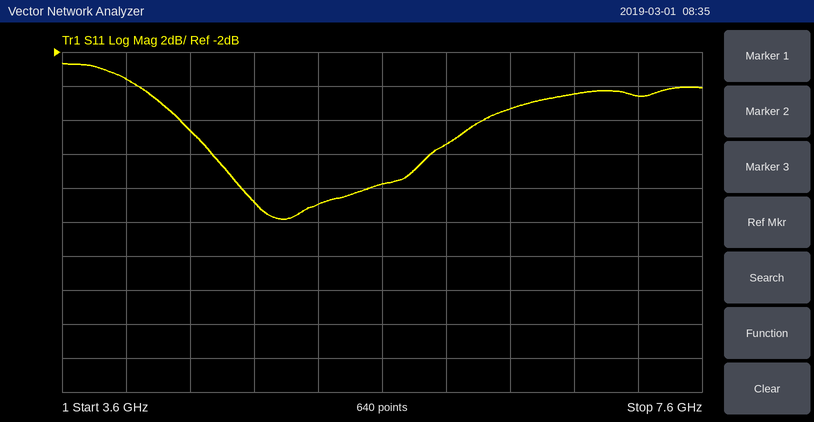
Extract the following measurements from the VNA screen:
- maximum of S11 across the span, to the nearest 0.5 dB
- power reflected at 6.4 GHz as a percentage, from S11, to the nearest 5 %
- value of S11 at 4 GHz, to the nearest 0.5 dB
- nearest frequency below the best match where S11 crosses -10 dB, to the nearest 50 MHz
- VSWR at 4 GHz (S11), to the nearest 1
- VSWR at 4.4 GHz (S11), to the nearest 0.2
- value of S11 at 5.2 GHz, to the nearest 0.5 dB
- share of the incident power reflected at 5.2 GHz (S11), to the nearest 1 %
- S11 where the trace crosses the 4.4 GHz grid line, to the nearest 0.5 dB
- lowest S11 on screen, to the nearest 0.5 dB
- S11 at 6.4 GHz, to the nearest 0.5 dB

-2.5 dB
30 %
-3.5 dB
4.70 GHz
5
2.8
-11.0 dB
8 %
-6.5 dB
-12.0 dB
-5.5 dB
